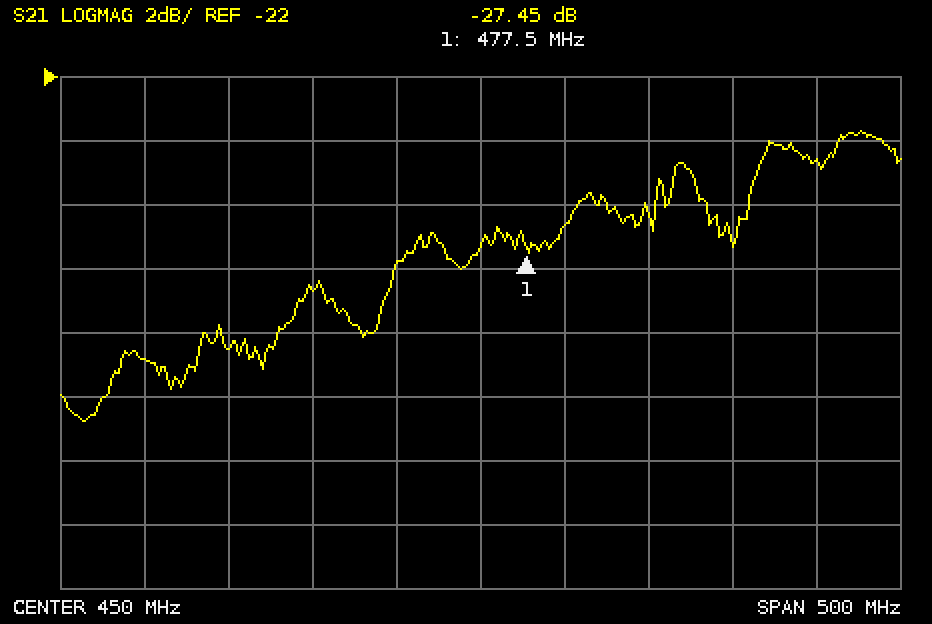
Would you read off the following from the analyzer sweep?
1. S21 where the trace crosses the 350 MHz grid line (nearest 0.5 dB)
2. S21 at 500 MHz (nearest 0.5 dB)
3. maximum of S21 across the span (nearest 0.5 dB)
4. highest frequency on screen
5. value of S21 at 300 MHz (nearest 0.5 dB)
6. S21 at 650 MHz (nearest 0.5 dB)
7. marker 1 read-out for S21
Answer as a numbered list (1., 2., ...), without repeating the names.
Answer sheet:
1. -28.5 dB
2. -26.5 dB
3. -23.5 dB
4. 700 MHz
5. -30.5 dB
6. -24.5 dB
7. -27.45 dB
